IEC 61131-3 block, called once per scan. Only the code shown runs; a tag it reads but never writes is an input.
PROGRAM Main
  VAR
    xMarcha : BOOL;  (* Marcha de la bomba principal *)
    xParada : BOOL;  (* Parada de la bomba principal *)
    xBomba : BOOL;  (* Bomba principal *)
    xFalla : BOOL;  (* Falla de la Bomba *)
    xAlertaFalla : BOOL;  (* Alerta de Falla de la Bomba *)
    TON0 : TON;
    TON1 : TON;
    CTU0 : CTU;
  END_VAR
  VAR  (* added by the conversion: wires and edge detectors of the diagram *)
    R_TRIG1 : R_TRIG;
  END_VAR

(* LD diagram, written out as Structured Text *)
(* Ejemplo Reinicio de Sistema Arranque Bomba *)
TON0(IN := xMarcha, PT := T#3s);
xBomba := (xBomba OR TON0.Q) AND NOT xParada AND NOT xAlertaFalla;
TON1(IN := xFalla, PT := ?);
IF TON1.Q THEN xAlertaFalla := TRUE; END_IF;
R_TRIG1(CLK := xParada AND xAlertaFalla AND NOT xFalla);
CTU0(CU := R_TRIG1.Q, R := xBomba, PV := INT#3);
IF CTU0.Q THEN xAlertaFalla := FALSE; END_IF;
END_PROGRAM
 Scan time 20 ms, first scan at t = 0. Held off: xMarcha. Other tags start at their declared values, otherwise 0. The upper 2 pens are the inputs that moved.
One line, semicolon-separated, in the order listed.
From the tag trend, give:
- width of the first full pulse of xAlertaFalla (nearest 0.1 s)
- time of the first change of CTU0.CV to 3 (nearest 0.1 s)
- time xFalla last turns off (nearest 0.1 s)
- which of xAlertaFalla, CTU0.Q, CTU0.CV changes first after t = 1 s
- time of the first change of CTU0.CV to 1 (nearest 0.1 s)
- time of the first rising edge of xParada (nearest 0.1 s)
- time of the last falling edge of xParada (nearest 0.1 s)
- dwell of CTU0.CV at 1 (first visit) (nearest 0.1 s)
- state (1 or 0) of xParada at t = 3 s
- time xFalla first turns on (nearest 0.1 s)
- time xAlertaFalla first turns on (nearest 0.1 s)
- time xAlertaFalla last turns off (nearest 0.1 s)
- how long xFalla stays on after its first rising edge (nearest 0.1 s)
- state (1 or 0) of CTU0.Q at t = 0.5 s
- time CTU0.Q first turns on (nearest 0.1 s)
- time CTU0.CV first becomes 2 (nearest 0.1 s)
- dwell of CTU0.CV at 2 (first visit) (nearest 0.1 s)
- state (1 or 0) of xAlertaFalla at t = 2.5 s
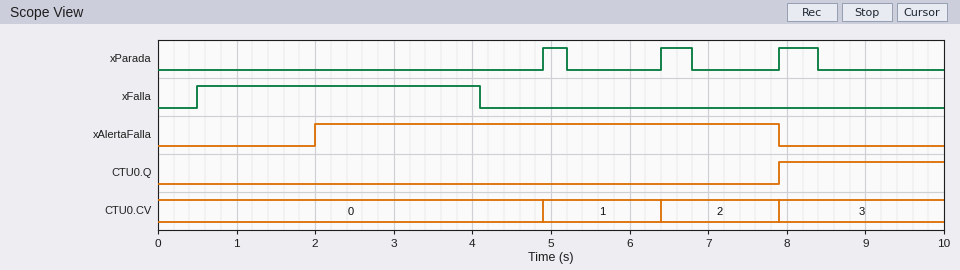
5.9 s; 7.9 s; 4.1 s; xAlertaFalla; 4.9 s; 4.9 s; 8.4 s; 1.5 s; 0; 0.5 s; 2.0 s; 7.9 s; 3.6 s; 0; 7.9 s; 6.4 s; 1.5 s; 1
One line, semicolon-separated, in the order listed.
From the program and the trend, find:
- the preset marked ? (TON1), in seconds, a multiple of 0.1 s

1.5 s
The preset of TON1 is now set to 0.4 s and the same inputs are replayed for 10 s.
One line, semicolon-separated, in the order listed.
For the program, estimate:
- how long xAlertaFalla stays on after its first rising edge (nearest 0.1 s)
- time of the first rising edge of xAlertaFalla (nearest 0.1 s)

7.0 s; 0.9 s
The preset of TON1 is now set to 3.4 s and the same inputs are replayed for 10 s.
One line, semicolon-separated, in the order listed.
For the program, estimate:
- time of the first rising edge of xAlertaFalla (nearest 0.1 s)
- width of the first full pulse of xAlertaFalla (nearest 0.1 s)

3.9 s; 4.0 s
